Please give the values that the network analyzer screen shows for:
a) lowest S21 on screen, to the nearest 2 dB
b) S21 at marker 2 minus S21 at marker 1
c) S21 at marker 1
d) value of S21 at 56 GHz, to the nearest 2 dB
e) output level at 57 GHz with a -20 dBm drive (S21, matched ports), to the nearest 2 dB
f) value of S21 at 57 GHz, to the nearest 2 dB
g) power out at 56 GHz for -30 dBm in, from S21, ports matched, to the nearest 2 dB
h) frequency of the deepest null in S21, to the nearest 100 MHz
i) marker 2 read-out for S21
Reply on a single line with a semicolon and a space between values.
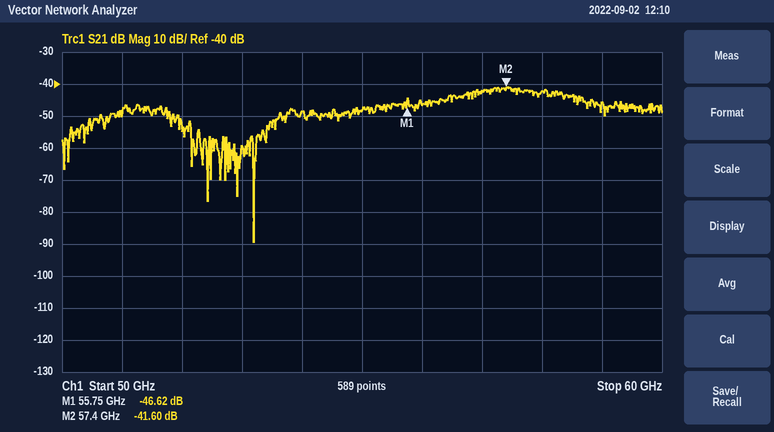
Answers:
-90 dB; 5.02 dB; -46.62 dB; -46 dB; -62 dBm; -42 dB; -76 dBm; 53.2 GHz; -41.60 dB
